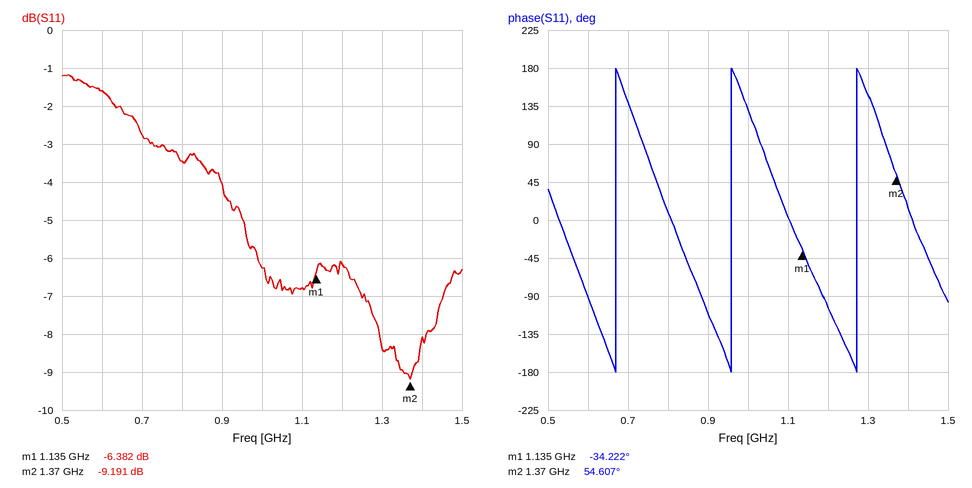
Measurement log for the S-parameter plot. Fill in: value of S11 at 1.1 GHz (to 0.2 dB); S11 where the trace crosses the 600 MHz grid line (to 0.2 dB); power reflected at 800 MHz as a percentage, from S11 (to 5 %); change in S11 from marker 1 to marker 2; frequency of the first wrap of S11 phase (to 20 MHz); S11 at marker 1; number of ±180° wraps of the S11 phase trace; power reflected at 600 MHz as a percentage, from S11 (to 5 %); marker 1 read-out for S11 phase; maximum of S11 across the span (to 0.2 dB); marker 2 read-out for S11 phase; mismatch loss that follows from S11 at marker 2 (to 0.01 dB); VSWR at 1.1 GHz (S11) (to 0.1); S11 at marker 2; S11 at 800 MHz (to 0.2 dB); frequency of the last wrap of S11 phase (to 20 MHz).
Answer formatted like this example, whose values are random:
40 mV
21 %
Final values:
-6.8 dB
-1.6 dB
45 %
-2.809 dB
660 MHz
-6.382 dB
3
70 %
-34.222°
-1.2 dB
54.607°
0.56 dB
2.7
-9.191 dB
-3.4 dB
1.28 GHz
